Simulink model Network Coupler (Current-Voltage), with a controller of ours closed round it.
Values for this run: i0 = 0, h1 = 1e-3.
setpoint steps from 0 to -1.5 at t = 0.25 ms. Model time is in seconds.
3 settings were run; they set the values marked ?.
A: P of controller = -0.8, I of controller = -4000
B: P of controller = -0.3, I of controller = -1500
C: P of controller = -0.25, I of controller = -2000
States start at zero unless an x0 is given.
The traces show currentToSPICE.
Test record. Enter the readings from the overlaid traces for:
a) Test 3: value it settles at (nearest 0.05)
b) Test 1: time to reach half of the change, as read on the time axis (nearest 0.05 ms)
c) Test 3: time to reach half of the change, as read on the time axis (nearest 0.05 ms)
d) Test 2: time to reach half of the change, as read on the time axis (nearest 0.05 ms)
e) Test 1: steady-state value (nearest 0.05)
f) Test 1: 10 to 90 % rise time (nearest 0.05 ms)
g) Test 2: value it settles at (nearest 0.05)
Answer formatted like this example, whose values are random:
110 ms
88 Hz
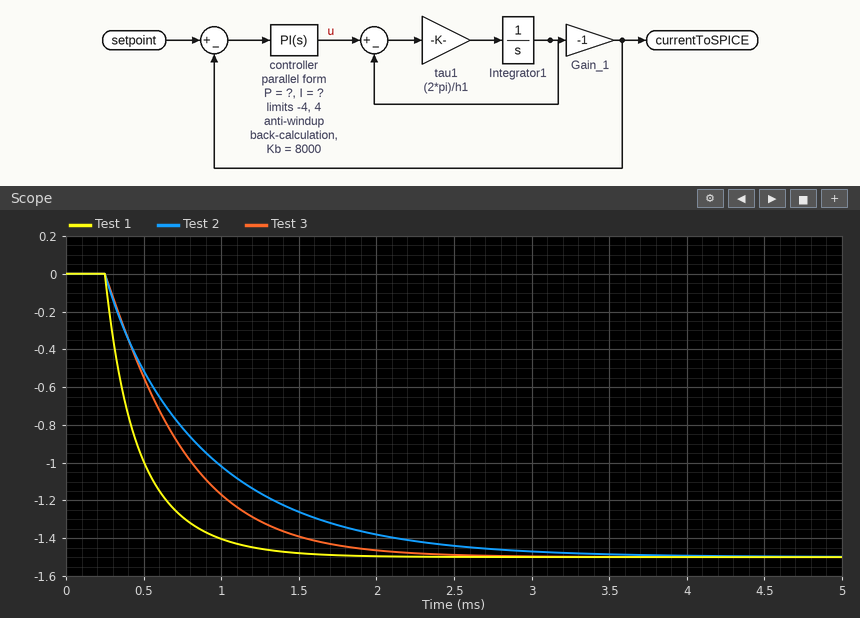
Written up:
-1.50
0.40 ms
0.60 ms
0.70 ms
-1.50
0.60 ms
-1.50
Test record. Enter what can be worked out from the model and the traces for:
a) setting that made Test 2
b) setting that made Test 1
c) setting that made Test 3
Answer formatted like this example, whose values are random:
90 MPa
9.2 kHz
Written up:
B
A
C
